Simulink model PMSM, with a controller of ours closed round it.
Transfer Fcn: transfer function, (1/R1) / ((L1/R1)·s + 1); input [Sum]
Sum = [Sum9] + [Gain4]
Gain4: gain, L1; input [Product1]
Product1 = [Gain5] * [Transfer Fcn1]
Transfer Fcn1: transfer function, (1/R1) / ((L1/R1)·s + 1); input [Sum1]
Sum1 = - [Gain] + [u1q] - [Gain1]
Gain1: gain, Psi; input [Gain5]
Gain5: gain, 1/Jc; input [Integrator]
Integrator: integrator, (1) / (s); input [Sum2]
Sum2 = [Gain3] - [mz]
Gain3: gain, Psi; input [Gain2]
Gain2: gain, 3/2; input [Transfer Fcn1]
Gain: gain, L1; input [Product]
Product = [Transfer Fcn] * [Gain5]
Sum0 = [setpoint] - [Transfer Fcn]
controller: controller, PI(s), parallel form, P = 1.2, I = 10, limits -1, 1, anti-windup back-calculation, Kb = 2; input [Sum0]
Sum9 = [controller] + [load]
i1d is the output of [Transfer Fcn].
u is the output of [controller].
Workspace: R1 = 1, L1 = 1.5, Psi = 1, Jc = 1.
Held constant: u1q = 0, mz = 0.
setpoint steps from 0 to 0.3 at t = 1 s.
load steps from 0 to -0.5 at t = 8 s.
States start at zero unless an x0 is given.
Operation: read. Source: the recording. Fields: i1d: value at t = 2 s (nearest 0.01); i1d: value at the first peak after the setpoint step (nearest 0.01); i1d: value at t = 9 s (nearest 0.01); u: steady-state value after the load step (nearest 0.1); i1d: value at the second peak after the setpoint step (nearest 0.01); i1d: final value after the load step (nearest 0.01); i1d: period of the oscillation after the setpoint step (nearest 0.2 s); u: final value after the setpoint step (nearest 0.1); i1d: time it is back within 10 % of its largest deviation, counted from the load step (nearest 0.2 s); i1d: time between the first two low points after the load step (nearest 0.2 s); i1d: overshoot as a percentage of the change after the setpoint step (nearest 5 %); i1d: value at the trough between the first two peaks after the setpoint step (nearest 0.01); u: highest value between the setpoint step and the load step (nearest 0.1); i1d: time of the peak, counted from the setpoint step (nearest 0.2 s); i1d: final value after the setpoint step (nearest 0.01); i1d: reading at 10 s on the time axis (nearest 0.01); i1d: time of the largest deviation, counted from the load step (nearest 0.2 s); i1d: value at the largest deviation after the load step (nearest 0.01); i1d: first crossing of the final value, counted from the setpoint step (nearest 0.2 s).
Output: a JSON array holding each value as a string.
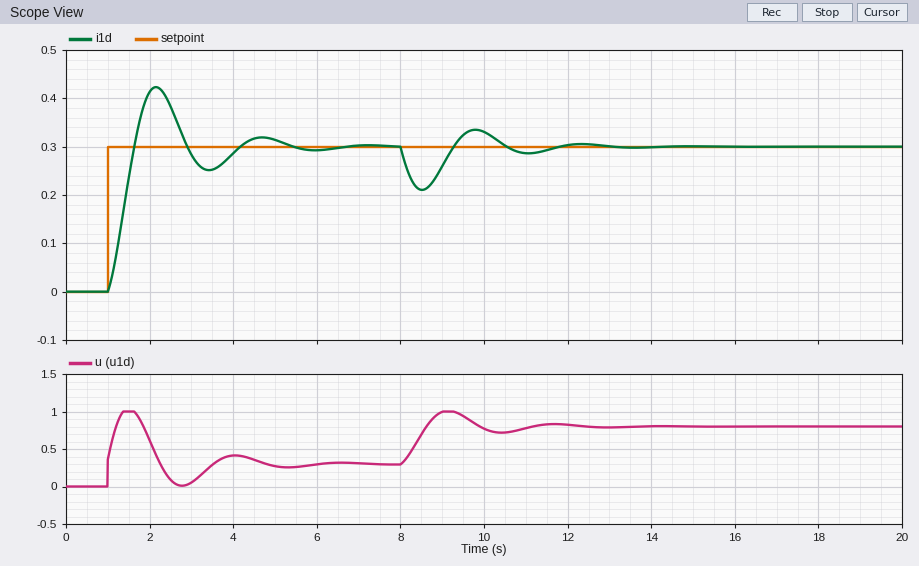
["0.41", "0.42", "0.26", "0.8", "0.32", "0.30", "2.6 s", "0.3", "3.4 s", "2.6 s", "40 %", "0.25", "1.0", "1.2 s", "0.30", "0.33", "0.6 s", "0.21", "0.6 s"]
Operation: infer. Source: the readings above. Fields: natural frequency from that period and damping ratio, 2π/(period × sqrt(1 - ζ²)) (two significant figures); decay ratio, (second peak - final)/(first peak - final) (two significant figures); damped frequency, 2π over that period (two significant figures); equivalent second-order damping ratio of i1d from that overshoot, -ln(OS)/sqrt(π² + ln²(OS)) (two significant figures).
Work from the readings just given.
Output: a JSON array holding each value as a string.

["2.5 rad/s", "0.17", "2.4 rad/s", "0.28"]
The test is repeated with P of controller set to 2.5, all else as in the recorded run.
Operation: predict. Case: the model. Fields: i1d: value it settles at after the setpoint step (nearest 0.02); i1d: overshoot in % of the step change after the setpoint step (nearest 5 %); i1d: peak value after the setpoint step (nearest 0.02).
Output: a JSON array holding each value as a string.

["0.30", "25 %", "0.38"]
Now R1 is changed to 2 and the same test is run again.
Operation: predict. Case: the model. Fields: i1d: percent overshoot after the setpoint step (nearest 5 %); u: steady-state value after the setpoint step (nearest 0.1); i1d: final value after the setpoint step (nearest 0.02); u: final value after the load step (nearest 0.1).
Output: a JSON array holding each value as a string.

["25 %", "0.6", "0.30", "1.0"]
